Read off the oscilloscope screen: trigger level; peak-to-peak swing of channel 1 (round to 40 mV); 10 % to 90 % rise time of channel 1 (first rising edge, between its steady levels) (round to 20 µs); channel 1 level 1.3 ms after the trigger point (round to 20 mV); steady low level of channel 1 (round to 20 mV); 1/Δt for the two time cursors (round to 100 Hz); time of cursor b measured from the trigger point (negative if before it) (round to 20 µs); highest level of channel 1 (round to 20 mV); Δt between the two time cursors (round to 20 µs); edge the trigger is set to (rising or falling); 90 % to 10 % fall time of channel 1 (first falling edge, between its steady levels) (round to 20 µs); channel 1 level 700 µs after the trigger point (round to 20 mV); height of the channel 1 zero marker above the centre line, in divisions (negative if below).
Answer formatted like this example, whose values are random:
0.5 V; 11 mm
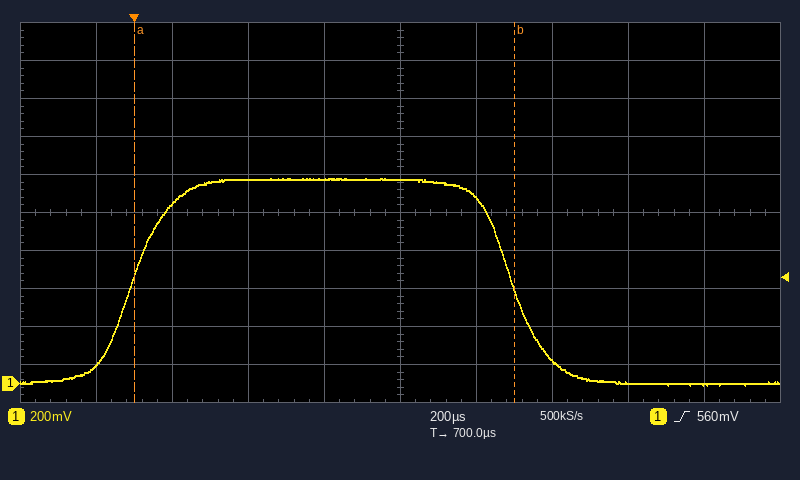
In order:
560 mV; 1.08 V; 200 µs; 0 mV; 0 mV; 1.0 kHz; +1.00 ms; 1.08 V; 1.00 ms; rising; 200 µs; 1.08 V; -4.5 div
